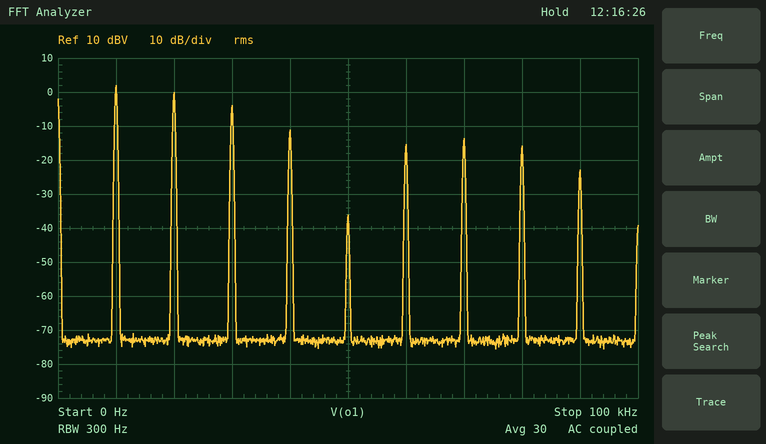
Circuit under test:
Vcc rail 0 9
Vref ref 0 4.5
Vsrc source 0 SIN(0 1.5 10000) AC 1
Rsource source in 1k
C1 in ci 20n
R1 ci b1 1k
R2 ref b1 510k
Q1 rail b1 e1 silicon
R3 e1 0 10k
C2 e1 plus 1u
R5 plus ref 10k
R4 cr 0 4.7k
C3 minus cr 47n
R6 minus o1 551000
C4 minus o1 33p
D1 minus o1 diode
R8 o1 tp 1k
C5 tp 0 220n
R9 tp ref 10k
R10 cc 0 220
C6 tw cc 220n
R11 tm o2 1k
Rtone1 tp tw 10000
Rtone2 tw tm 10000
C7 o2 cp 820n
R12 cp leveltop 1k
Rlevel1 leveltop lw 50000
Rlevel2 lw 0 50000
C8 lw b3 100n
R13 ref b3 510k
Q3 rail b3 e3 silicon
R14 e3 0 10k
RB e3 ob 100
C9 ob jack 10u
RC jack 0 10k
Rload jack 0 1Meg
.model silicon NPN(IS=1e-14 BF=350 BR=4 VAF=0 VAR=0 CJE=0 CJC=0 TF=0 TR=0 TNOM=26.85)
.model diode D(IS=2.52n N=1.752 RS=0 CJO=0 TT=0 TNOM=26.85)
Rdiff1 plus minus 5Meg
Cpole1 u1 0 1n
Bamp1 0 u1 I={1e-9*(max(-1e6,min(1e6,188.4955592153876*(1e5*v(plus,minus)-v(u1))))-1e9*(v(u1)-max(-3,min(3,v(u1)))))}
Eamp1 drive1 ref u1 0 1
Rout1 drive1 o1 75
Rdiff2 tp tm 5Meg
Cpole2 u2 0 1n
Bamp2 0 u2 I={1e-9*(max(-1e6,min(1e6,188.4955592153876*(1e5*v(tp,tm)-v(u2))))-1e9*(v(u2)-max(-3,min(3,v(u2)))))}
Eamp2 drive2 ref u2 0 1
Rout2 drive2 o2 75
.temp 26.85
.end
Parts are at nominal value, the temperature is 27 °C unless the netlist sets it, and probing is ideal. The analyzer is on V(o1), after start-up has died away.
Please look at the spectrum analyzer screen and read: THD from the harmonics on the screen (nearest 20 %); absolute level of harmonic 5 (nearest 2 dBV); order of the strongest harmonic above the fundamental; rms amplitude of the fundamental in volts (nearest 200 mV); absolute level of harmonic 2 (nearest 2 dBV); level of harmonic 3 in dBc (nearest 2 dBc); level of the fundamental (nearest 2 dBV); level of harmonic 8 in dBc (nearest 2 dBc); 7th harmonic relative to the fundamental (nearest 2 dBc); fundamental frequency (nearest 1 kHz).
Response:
100 %
-36 dBV
2
1.2 V
0 dBV
-6 dBc
2 dBV
-18 dBc
-16 dBc
10 kHz
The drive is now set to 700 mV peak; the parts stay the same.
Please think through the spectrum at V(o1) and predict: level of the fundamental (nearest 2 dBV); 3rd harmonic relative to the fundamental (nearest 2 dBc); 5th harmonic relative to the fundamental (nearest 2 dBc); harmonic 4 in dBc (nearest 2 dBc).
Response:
2 dBV
-8 dBc
-18 dBc
-26 dBc
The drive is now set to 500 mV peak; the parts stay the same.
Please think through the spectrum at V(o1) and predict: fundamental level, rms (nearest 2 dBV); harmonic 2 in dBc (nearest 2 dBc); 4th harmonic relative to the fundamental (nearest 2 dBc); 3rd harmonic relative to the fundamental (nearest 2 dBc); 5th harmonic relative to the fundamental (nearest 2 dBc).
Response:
2 dBV
-4 dBc
-28 dBc
-12 dBc
-16 dBc
